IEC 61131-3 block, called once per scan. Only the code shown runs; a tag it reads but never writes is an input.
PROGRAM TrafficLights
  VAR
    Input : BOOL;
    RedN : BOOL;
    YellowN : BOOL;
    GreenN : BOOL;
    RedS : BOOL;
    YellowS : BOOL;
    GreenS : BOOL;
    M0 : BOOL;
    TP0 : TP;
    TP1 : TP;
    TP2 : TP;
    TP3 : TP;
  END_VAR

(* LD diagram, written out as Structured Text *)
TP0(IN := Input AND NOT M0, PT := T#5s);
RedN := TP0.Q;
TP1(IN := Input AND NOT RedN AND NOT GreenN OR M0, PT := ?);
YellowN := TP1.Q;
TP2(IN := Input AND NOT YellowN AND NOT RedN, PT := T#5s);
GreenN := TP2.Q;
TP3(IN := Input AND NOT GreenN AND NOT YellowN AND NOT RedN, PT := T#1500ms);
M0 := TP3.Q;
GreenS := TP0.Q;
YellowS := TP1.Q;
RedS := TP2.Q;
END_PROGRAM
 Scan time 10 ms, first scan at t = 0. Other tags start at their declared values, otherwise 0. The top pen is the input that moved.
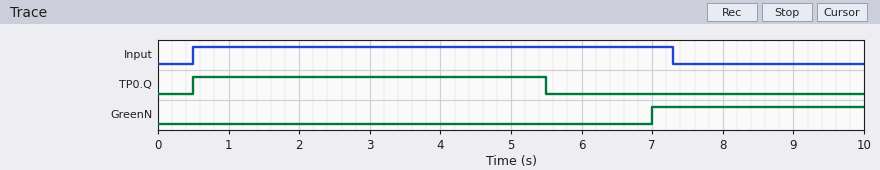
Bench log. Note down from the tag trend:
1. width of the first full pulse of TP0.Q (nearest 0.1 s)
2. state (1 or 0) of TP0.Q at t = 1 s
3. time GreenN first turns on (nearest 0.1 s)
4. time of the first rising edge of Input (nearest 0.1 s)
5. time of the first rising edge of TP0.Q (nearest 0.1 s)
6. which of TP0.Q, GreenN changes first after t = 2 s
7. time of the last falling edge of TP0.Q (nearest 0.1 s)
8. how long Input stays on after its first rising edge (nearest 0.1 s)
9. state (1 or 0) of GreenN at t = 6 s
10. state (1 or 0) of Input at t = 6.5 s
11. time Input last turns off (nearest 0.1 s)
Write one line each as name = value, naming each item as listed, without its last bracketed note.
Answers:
width of the first full pulse of TP0.Q = 5.0 s
state (1 or 0) of TP0.Q at t = 1 s = 1
time GreenN first turns on = 7.0 s
time of the first rising edge of Input = 0.5 s
time of the first rising edge of TP0.Q = 0.5 s
which of TP0.Q, GreenN changes first after t = 2 s = TP0.Q
time of the last falling edge of TP0.Q = 5.5 s
how long Input stays on after its first rising edge = 6.8 s
state (1 or 0) of GreenN at t = 6 s = 0
state (1 or 0) of Input at t = 6.5 s = 1
time Input last turns off = 7.3 s
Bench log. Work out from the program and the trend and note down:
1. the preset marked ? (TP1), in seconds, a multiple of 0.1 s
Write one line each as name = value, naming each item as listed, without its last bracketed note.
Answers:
the preset marked ? (TP1), in seconds, a multiple of 0.1 s = 1.5 s
